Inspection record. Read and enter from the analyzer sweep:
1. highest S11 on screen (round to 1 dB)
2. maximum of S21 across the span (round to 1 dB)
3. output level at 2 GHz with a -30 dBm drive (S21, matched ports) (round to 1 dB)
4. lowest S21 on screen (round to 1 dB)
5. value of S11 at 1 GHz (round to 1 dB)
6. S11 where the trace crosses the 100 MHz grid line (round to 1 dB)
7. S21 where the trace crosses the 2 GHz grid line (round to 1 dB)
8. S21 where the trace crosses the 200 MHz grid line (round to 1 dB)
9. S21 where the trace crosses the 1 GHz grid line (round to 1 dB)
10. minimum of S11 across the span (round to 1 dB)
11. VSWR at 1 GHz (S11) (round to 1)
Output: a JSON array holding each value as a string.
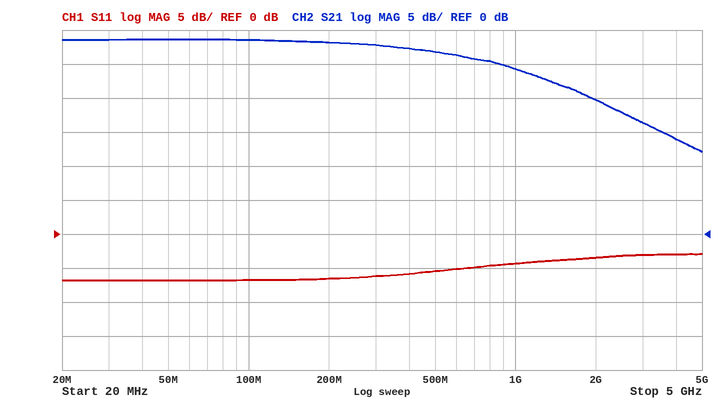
["-3 dB", "29 dB", "-10 dBm", "12 dB", "-4 dB", "-7 dB", "20 dB", "28 dB", "24 dB", "-7 dB", "4"]
